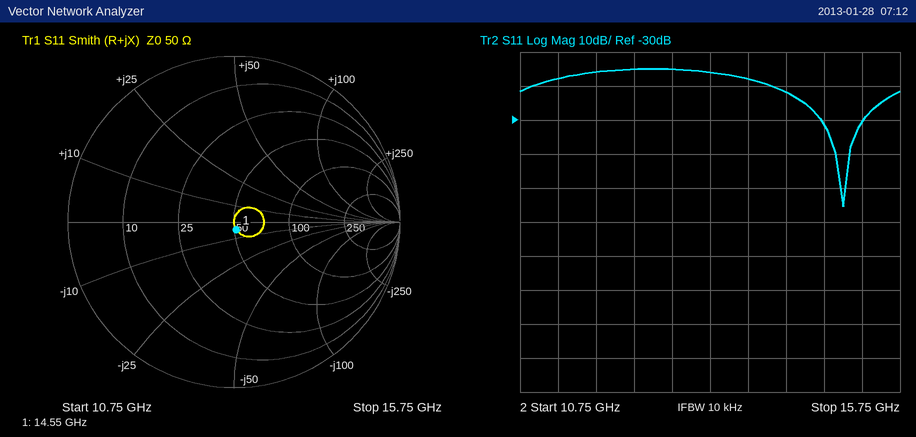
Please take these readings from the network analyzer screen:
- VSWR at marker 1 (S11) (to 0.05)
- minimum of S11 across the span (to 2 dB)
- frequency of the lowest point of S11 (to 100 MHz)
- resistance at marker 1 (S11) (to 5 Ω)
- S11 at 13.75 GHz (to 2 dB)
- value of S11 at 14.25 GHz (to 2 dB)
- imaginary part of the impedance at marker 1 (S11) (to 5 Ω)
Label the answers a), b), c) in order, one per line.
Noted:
a) 1.10
b) -56 dB
c) 15.0 GHz
d) 50 Ω
e) -18 dB
f) -22 dB
g) -5 Ω
